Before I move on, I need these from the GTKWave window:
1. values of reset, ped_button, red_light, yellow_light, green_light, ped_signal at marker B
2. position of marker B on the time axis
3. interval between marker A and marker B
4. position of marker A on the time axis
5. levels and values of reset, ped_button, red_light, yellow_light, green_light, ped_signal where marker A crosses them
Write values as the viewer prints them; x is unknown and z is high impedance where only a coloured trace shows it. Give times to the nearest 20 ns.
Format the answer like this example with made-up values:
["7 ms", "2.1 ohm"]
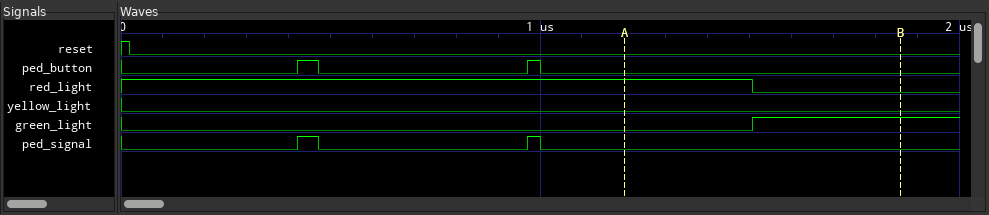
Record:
["reset=0, ped_button=0, red_light=0, yellow_light=0, green_light=1, ped_signal=0", "1860 ns", "660 ns", "1200 ns", "reset=0, ped_button=0, red_light=1, yellow_light=0, green_light=0, ped_signal=0"]
